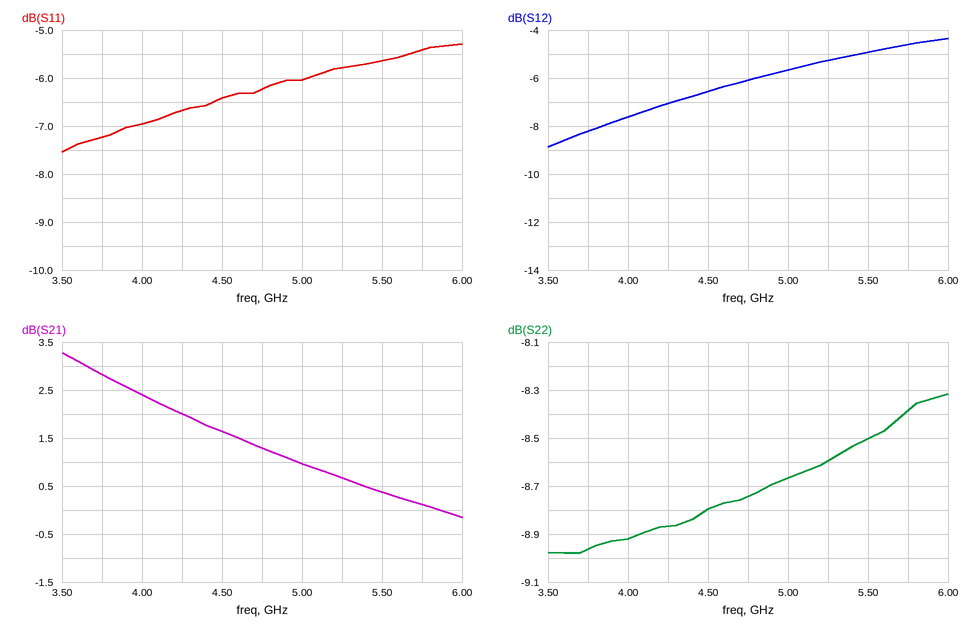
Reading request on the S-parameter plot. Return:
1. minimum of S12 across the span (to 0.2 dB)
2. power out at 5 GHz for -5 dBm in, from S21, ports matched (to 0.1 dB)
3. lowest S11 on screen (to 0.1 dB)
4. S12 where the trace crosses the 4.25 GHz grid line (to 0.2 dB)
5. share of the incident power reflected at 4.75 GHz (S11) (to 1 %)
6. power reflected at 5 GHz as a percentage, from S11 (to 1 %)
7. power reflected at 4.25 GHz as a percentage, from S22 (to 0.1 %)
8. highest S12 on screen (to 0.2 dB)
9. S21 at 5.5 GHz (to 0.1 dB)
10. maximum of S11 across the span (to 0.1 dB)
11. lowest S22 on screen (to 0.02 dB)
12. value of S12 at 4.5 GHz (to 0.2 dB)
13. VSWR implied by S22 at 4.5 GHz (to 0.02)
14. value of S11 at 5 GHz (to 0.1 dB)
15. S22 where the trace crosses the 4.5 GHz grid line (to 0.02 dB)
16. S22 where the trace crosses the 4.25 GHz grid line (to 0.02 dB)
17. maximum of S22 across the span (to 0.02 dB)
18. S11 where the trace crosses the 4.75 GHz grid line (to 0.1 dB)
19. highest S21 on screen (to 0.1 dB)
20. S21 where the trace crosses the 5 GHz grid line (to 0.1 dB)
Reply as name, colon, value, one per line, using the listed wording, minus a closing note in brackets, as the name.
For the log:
minimum of S12 across the span: -8.8 dB
power out at 5 GHz for -5 dBm in, from S21, ports matched: -4.0 dBm
lowest S11 on screen: -7.5 dB
S12 where the trace crosses the 4.25 GHz grid line: -7.0 dB
share of the incident power reflected at 4.75 GHz (S11): 24 %
power reflected at 5 GHz as a percentage, from S11: 25 %
power reflected at 4.25 GHz as a percentage, from S22: 13.0 %
highest S12 on screen: -4.4 dB
S21 at 5.5 GHz: 0.4 dB
maximum of S11 across the span: -5.3 dB
lowest S22 on screen: -8.98 dB
value of S12 at 4.5 GHz: -6.6 dB
VSWR implied by S22 at 4.5 GHz: 2.14
value of S11 at 5 GHz: -6.0 dB
S22 where the trace crosses the 4.5 GHz grid line: -8.80 dB
S22 where the trace crosses the 4.25 GHz grid line: -8.86 dB
maximum of S22 across the span: -8.32 dB
S11 where the trace crosses the 4.75 GHz grid line: -6.2 dB
highest S21 on screen: 3.3 dB
S21 where the trace crosses the 5 GHz grid line: 1.0 dB
